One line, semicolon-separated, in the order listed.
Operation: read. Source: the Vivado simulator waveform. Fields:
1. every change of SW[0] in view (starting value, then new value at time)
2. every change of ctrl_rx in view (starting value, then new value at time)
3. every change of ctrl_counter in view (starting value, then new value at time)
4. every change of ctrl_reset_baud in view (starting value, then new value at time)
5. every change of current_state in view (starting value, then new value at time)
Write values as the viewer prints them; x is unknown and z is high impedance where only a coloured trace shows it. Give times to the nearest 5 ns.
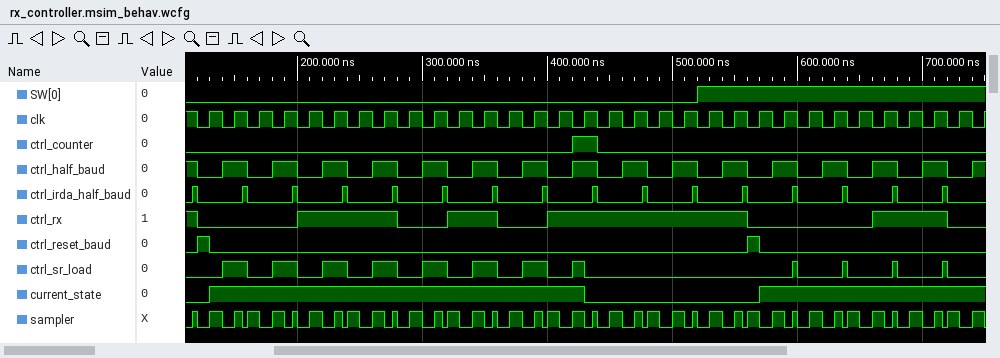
0, 1 at 520 ns; 1, 0 at 120 ns, 1 at 200 ns, 0 at 280 ns, 1 at 320 ns, 0 at 360 ns, 1 at 400 ns, 0 at 560 ns, 1 at 660 ns, 0 at 720 ns; 0, 1 at 420 ns, 0 at 440 ns; 0, 1 at 120 ns, 0 at 130 ns, 1 at 560 ns, 0 at 570 ns; 0, 1 at 130 ns, 0 at 430 ns, 1 at 570 ns
